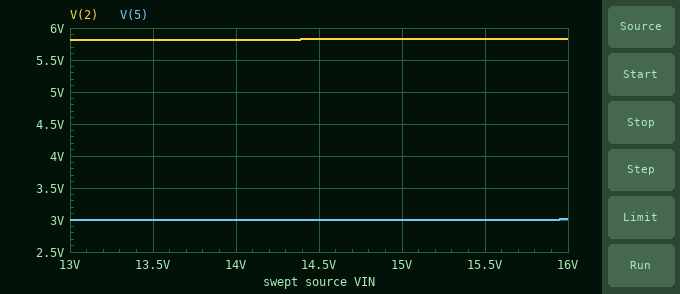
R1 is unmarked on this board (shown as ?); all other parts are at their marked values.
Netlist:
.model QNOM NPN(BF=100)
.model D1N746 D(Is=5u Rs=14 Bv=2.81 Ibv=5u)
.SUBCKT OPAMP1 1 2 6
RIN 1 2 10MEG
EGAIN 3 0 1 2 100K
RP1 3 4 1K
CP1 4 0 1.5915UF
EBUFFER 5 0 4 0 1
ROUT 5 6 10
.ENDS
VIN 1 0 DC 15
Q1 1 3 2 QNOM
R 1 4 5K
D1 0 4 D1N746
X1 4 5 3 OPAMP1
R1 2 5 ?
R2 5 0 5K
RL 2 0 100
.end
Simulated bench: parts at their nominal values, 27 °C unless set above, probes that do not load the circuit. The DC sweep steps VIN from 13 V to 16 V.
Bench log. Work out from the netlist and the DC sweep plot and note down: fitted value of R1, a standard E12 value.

4.7 kΩ
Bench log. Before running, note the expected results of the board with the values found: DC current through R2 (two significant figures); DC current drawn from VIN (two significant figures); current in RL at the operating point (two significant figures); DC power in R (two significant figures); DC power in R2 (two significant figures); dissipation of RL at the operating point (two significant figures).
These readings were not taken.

600 µA
61 mA
58 mA
29 mW
1.8 mW
340 mW
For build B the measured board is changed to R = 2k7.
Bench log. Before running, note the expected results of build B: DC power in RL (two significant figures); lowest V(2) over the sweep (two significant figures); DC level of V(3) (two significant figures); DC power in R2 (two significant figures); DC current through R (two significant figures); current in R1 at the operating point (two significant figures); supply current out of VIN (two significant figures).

350 mW
5.9 V
6.8 V
1.9 mW
4.4 mA
610 µA
64 mA
